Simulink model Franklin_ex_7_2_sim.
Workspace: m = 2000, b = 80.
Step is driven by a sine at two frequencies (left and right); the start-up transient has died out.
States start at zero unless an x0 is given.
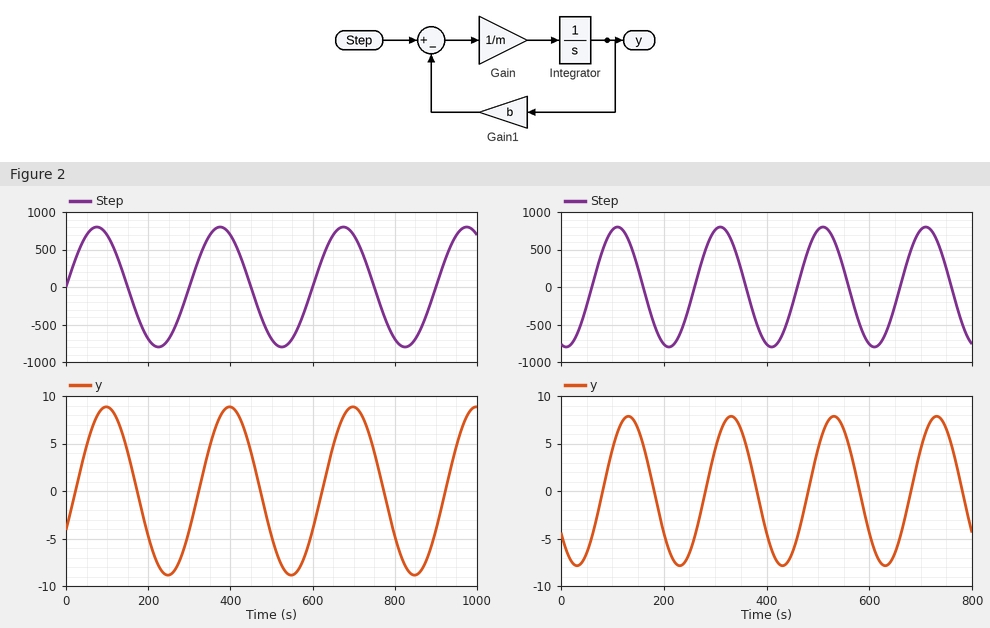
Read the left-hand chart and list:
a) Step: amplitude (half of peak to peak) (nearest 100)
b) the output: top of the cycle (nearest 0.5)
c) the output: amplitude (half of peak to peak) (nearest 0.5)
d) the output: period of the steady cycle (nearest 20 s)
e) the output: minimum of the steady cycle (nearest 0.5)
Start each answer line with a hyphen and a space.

- 800
- 9.0
- 9.0
- 300 s
- -9.0
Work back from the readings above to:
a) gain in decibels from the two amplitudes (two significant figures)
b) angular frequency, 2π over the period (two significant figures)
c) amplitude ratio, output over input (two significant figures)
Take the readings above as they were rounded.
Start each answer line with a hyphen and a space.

- -39 dB
- 0.021 rad/s
- 0.011
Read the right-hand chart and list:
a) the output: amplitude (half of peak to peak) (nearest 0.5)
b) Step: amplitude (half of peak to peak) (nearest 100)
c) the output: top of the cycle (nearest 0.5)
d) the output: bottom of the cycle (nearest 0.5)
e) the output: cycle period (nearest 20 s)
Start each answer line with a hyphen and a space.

- 8.0
- 800
- 8.0
- -8.0
- 200 s
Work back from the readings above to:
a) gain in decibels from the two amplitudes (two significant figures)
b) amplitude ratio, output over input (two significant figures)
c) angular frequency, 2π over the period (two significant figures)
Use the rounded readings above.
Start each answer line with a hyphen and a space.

- -40 dB
- 0.010
- 0.031 rad/s
